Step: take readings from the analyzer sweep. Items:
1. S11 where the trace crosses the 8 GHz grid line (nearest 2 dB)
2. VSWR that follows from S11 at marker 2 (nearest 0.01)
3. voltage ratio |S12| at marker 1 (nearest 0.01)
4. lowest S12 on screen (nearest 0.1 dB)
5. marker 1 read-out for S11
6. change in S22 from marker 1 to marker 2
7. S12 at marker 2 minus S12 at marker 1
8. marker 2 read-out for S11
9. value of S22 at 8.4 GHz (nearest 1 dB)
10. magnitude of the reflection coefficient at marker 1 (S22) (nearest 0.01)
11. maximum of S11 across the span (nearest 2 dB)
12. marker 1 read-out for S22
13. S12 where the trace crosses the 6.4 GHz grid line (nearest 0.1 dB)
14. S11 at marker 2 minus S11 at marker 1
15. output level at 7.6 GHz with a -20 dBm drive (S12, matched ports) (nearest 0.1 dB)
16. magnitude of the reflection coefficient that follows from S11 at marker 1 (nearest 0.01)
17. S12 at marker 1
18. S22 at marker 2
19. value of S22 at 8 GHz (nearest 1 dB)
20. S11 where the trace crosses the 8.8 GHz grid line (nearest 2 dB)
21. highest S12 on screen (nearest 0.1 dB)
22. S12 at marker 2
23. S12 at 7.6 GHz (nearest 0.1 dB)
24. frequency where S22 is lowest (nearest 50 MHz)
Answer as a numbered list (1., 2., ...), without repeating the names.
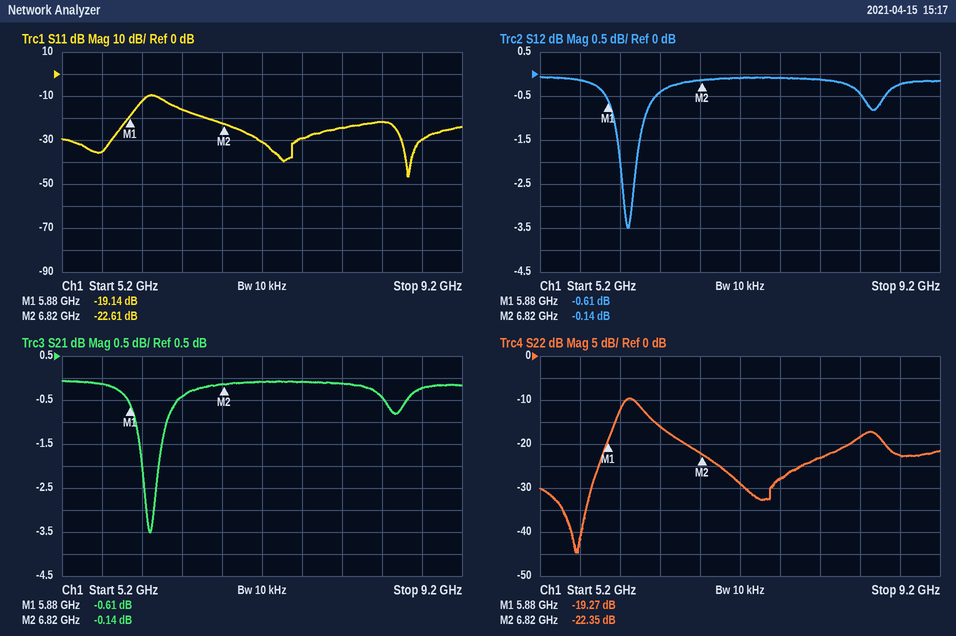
1. -24 dB
2. 1.16
3. 0.93
4. -3.5 dB
5. -19.14 dB
6. -3.08 dB
7. 0.47 dB
8. -22.61 dB
9. -18 dB
10. 0.11
11. -10 dB
12. -19.27 dB
13. -0.4 dB
14. -3.47 dB
15. -20.1 dBm
16. 0.11
17. -0.61 dB
18. -22.35 dB
19. -23 dB
20. -30 dB
21. -0.1 dB
22. -0.14 dB
23. -0.1 dB
24. 5.55 GHz
